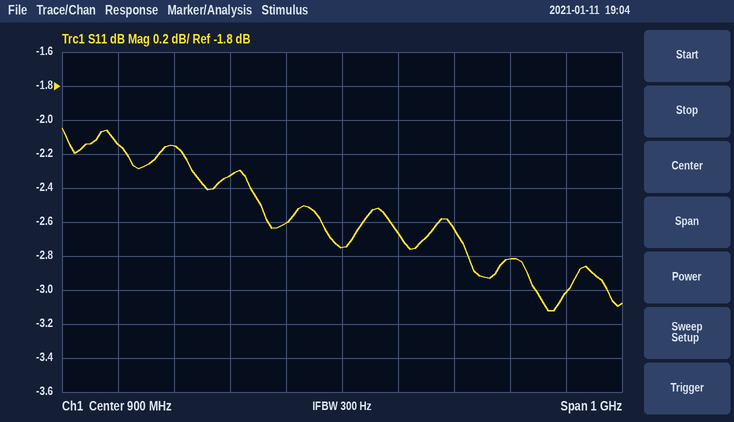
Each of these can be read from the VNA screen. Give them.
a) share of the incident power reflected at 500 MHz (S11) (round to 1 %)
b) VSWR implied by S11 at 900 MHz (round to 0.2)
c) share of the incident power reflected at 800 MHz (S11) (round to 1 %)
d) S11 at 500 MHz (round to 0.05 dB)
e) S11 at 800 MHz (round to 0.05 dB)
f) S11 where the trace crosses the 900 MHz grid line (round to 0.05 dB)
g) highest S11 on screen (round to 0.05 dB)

61 %
6.4
55 %
-2.15 dB
-2.60 dB
-2.75 dB
-2.05 dB
